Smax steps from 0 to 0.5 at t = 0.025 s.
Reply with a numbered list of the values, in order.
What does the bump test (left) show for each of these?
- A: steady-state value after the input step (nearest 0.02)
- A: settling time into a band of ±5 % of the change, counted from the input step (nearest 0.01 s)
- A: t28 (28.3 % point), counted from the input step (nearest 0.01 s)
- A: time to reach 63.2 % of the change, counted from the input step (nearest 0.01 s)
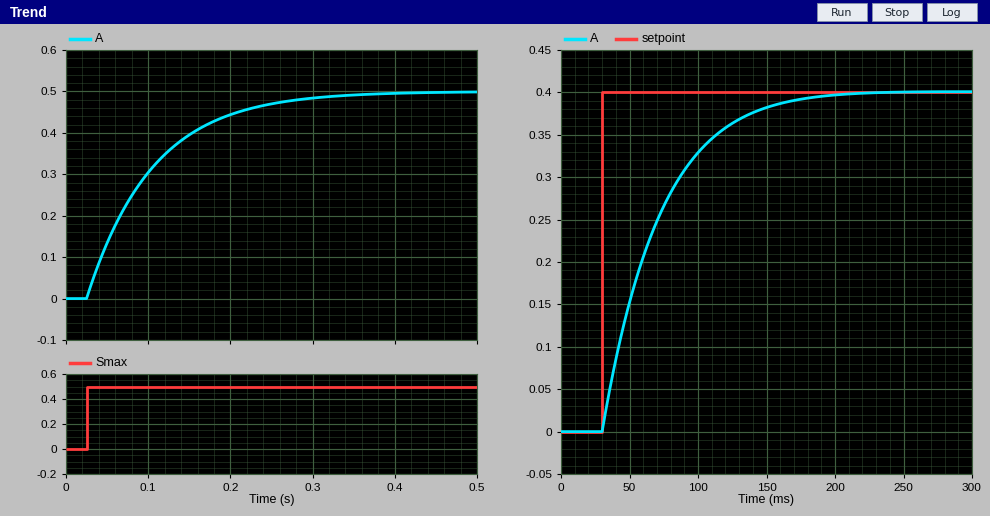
1. 0.50
2. 0.24 s
3. 0.03 s
4. 0.08 s
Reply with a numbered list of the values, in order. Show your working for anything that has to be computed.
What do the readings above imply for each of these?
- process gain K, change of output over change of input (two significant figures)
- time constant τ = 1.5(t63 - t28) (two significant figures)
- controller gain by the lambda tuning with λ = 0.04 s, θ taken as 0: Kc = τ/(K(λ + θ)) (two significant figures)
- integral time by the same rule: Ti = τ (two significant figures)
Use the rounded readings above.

1. (0.5 - 0) / 0.5 = 1.0
2. 1.5 × (0.08 - 0.03) = 0.075 s
3. 0.075 / (1 × (0.04 + 0)) = 1.9
4. 0.075 s
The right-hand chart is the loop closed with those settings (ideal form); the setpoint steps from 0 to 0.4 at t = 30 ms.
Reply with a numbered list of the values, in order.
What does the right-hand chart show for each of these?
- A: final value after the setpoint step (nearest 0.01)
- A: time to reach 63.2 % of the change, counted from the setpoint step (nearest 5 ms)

1. 0.40
2. 40 ms
